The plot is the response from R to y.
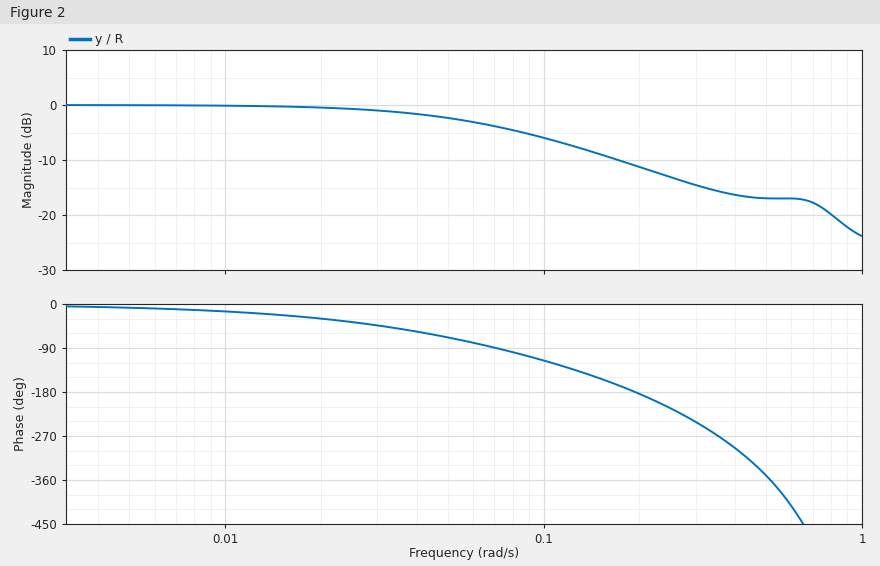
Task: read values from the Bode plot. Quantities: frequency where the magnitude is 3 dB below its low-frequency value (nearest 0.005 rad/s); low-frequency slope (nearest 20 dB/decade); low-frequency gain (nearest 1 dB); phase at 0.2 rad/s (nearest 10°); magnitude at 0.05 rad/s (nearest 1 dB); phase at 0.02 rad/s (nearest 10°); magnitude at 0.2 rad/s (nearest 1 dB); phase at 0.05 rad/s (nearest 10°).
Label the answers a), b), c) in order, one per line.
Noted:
a) 0.060 rad/s
b) 0 dB/decade
c) 0 dB
d) -180°
e) -2 dB
f) -30°
g) -11 dB
h) -70°
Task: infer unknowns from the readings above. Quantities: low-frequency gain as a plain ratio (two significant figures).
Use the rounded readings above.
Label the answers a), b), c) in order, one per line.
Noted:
a) 1.0
